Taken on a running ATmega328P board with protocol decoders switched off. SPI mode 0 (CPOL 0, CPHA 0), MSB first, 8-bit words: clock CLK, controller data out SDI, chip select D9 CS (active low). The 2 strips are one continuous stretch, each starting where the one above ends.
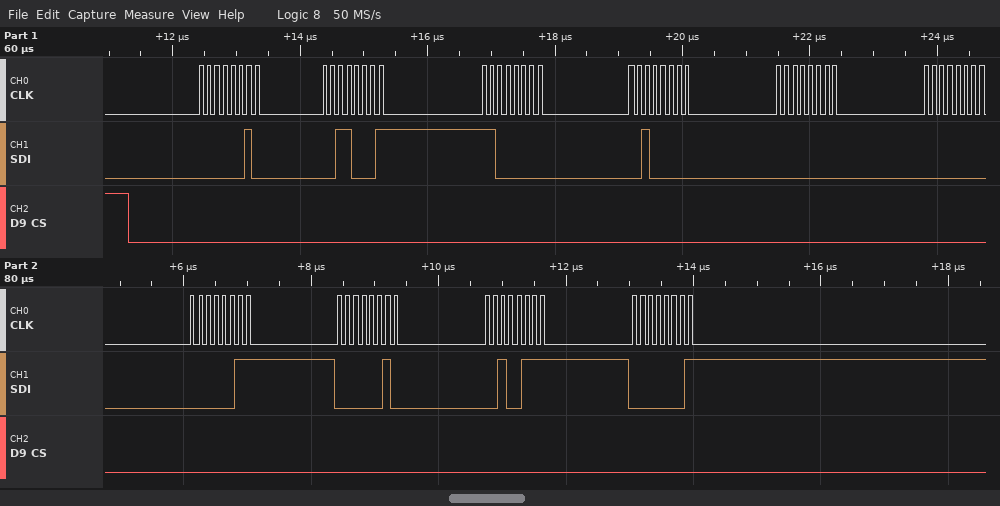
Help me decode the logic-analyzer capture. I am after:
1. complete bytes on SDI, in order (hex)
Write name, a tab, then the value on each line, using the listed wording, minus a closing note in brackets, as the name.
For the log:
complete bytes on SDI, in order	0x02 0x31 0xC0 0x20 0x00 0x00 0x03 0x02 0x27 0x01
